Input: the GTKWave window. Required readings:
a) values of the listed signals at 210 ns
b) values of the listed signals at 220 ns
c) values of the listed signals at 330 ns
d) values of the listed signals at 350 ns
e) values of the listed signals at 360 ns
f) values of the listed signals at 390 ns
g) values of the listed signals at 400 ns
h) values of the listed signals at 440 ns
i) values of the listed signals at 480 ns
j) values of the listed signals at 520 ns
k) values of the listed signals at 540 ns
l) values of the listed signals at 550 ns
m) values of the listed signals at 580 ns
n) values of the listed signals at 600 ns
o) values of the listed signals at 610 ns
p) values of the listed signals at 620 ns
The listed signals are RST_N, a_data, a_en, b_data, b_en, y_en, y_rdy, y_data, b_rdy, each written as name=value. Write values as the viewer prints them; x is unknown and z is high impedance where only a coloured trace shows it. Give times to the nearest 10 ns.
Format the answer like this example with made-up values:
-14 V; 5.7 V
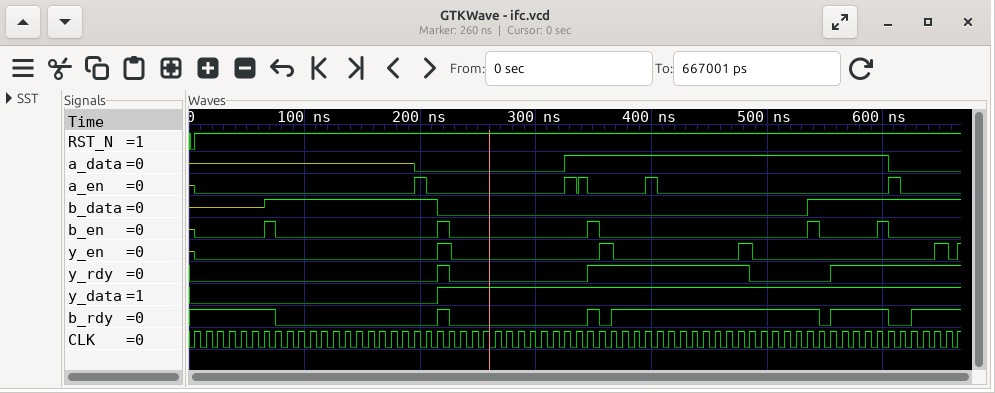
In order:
RST_N=1, a_data=0, a_en=0, b_data=1, b_en=0, y_en=0, y_rdy=0, y_data=0, b_rdy=0; RST_N=1, a_data=0, a_en=0, b_data=0, b_en=1, y_en=1, y_rdy=1, y_data=1, b_rdy=1; RST_N=1, a_data=1, a_en=1, b_data=0, b_en=0, y_en=0, y_rdy=0, y_data=1, b_rdy=0; RST_N=1, a_data=1, a_en=0, b_data=0, b_en=1, y_en=0, y_rdy=1, y_data=1, b_rdy=1; RST_N=1, a_data=1, a_en=0, b_data=0, b_en=0, y_en=1, y_rdy=1, y_data=1, b_rdy=0; RST_N=1, a_data=1, a_en=0, b_data=0, b_en=0, y_en=0, y_rdy=1, y_data=1, b_rdy=1; RST_N=1, a_data=1, a_en=1, b_data=0, b_en=0, y_en=0, y_rdy=1, y_data=1, b_rdy=1; RST_N=1, a_data=1, a_en=0, b_data=0, b_en=0, y_en=0, y_rdy=1, y_data=1, b_rdy=1; RST_N=1, a_data=1, a_en=0, b_data=0, b_en=0, y_en=1, y_rdy=1, y_data=1, b_rdy=1; RST_N=1, a_data=1, a_en=0, b_data=0, b_en=0, y_en=0, y_rdy=0, y_data=1, b_rdy=1; RST_N=1, a_data=1, a_en=0, b_data=1, b_en=1, y_en=0, y_rdy=0, y_data=1, b_rdy=1; RST_N=1, a_data=1, a_en=0, b_data=1, b_en=0, y_en=0, y_rdy=0, y_data=1, b_rdy=0; RST_N=1, a_data=1, a_en=0, b_data=1, b_en=0, y_en=0, y_rdy=1, y_data=1, b_rdy=1; RST_N=1, a_data=1, a_en=0, b_data=1, b_en=1, y_en=0, y_rdy=1, y_data=1, b_rdy=1; RST_N=1, a_data=0, a_en=1, b_data=1, b_en=0, y_en=0, y_rdy=1, y_data=1, b_rdy=0; RST_N=1, a_data=0, a_en=0, b_data=1, b_en=0, y_en=0, y_rdy=1, y_data=1, b_rdy=0
